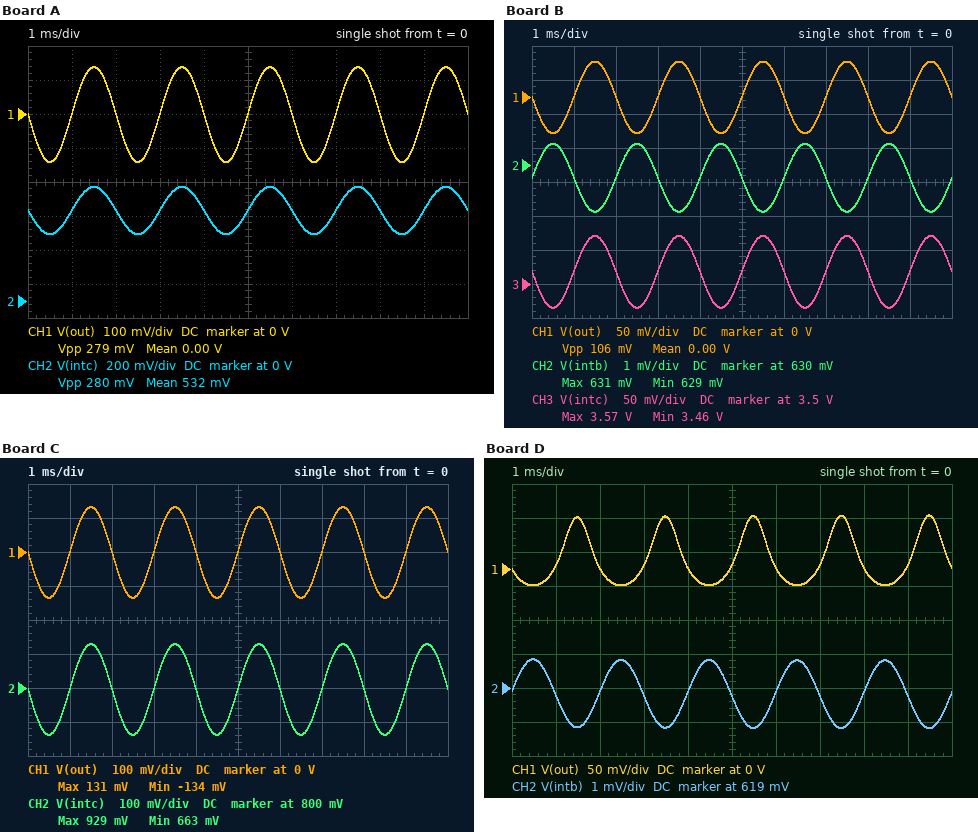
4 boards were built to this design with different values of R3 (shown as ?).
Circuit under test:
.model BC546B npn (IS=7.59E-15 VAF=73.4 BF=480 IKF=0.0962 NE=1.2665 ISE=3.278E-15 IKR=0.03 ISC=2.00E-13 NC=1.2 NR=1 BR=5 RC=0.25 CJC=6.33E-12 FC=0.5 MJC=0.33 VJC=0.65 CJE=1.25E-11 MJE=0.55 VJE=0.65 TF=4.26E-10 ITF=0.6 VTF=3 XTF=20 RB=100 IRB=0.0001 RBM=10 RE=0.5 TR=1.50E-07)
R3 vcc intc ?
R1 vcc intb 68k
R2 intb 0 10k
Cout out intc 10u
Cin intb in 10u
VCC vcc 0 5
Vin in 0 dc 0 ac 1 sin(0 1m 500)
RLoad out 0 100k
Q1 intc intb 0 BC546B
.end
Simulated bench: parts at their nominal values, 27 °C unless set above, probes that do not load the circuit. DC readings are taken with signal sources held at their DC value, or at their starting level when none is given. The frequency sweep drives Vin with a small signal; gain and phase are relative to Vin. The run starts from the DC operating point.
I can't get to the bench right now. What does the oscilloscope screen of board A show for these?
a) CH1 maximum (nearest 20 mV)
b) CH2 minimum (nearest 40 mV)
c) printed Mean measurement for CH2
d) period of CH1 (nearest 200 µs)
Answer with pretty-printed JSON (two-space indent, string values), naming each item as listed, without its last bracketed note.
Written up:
{
  "CH1 maximum": "140 mV",
  "CH2 minimum": "400 mV",
  "printed Mean measurement for CH2": "532 mV",
  "period of CH1": "2.0 ms"
}
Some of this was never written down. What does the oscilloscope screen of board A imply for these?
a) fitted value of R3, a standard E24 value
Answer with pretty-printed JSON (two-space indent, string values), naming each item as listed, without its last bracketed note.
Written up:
{
  "fitted value of R3, a standard E24 value": "16 kΩ"
}
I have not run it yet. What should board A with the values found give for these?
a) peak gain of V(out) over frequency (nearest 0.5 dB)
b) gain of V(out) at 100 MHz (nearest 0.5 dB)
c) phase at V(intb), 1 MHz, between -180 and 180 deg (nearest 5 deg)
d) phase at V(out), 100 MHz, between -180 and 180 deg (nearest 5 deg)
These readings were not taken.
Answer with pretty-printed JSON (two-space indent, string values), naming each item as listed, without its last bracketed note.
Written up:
{
  "peak gain of V(out) over frequency": "43.0 dB",
  "gain of V(out) at 100 MHz": "-0.5 dB",
  "phase at V(intb), 1 MHz, between -180 and 180 deg": "0 deg",
  "phase at V(out), 100 MHz, between -180 and 180 deg": "25 deg"
}
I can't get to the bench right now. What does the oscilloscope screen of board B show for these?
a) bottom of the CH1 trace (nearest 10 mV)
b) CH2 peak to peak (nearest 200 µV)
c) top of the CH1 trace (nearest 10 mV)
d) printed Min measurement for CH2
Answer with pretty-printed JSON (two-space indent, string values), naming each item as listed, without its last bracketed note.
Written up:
{
  "bottom of the CH1 trace": "-50 mV",
  "CH2 peak to peak": "2.0 mV",
  "top of the CH1 trace": "50 mV",
  "printed Min measurement for CH2": "629 mV"
}
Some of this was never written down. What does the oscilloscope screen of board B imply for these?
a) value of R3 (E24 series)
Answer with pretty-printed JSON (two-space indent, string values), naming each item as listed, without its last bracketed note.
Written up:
{
  "value of R3": "5.1 kΩ"
}
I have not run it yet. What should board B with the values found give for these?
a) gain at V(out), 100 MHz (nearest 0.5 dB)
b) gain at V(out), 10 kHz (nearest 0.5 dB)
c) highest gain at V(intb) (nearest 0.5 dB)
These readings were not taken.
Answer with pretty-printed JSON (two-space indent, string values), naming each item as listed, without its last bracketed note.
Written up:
{
  "gain at V(out), 100 MHz": "4.5 dB",
  "gain at V(out), 10 kHz": "34.5 dB",
  "highest gain at V(intb)": "0 dB"
}
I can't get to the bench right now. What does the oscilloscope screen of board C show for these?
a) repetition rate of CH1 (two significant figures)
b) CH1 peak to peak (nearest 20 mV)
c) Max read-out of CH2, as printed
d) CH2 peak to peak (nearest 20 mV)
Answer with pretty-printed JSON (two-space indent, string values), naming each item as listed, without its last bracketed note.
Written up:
{
  "repetition rate of CH1": "500 Hz",
  "CH1 peak to peak": "260 mV",
  "Max read-out of CH2, as printed": "929 mV",
  "CH2 peak to peak": "260 mV"
}
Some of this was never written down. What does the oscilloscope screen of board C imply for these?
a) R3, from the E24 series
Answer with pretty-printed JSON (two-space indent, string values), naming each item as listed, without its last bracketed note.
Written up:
{
  "R3, from the E24 series": "15 kΩ"
}
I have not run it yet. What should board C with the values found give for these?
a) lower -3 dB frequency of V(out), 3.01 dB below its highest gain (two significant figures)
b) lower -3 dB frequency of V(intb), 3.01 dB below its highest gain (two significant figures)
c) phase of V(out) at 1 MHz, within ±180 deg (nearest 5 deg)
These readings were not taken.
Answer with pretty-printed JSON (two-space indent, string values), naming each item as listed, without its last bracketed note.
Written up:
{
  "lower -3 dB frequency of V(out), 3.01 dB below its highest gain": "2.5 Hz",
  "lower -3 dB frequency of V(intb), 3.01 dB below its highest gain": "2.5 Hz",
  "phase of V(out) at 1 MHz, within ±180 deg": "135 deg"
}
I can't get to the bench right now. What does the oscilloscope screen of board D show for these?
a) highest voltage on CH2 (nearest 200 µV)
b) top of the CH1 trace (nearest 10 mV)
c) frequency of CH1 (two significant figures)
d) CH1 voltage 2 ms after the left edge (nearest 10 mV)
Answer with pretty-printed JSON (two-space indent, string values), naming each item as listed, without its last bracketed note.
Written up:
{
  "highest voltage on CH2": "619.8 mV",
  "top of the CH1 trace": "80 mV",
  "frequency of CH1": "500 Hz",
  "CH1 voltage 2 ms after the left edge": "0 V"
}
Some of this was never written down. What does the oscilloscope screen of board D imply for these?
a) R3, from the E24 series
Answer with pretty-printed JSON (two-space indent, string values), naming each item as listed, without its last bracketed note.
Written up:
{
  "R3, from the E24 series": "27 kΩ"
}
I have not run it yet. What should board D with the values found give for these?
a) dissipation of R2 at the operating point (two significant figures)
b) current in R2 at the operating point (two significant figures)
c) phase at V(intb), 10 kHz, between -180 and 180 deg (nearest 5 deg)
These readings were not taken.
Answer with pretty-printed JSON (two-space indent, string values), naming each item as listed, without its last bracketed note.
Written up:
{
  "dissipation of R2 at the operating point": "38 µW",
  "current in R2 at the operating point": "62 µA",
  "phase at V(intb), 10 kHz, between -180 and 180 deg": "0 deg"
}
